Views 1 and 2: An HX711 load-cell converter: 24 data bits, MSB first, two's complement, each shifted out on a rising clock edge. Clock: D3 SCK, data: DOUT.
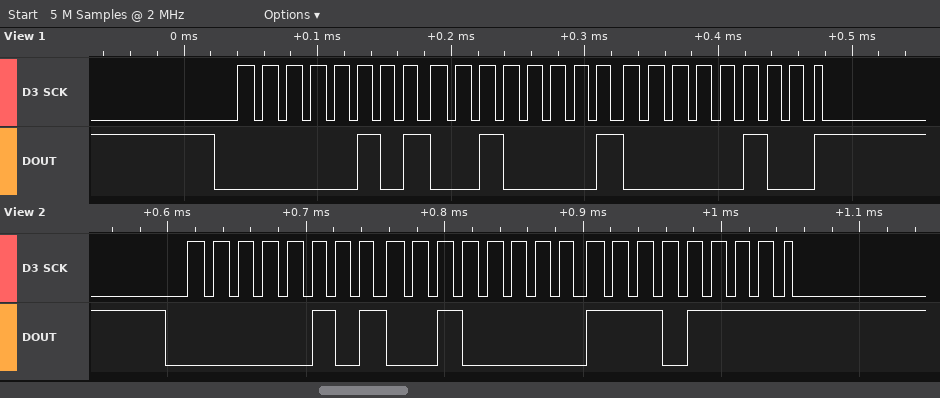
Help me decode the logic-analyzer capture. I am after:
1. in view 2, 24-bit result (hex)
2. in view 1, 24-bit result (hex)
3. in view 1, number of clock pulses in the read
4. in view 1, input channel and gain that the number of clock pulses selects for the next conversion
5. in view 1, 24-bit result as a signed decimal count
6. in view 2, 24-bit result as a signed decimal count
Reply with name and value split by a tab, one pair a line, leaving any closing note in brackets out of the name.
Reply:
in view 2, 24-bit result	0x0520EF
in view 1, 24-bit result	0x052104
in view 1, number of clock pulses in the read	25
in view 1, input channel and gain that the number of clock pulses selects for the next conversion	channel A, gain 128
in view 1, 24-bit result as a signed decimal count	336132
in view 2, 24-bit result as a signed decimal count	336111
